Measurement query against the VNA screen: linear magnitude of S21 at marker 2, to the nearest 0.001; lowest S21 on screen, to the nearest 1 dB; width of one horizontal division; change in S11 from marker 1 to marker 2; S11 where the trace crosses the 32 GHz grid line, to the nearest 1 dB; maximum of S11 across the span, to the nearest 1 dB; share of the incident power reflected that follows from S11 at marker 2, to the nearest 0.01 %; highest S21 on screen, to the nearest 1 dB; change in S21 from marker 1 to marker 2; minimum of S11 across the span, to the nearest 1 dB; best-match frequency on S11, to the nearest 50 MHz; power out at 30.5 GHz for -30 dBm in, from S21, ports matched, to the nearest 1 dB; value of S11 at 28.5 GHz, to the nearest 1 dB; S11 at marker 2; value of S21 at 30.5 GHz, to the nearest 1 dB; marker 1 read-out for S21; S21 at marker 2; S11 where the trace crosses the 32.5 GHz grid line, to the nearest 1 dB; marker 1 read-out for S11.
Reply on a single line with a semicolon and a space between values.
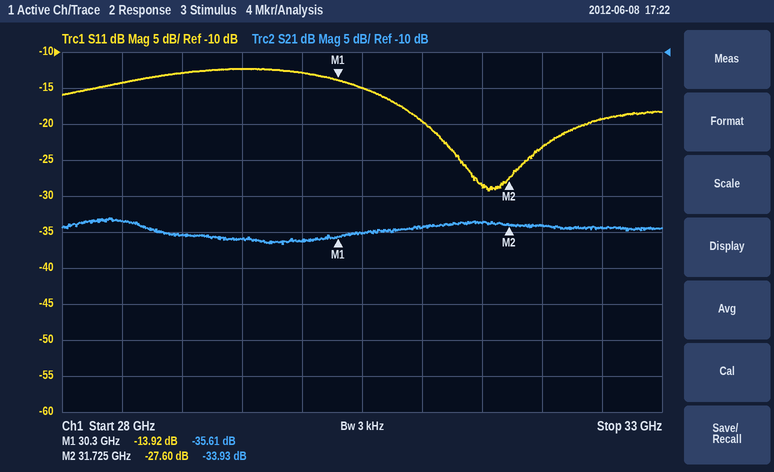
0.020; -37 dB; 500 MHz; -13.68 dB; -23 dB; -12 dB; 0.17 %; -33 dB; 1.68 dB; -29 dB; 31.55 GHz; -65 dBm; -14 dB; -27.60 dB; -35 dB; -35.61 dB; -33.93 dB; -19 dB; -13.92 dB
